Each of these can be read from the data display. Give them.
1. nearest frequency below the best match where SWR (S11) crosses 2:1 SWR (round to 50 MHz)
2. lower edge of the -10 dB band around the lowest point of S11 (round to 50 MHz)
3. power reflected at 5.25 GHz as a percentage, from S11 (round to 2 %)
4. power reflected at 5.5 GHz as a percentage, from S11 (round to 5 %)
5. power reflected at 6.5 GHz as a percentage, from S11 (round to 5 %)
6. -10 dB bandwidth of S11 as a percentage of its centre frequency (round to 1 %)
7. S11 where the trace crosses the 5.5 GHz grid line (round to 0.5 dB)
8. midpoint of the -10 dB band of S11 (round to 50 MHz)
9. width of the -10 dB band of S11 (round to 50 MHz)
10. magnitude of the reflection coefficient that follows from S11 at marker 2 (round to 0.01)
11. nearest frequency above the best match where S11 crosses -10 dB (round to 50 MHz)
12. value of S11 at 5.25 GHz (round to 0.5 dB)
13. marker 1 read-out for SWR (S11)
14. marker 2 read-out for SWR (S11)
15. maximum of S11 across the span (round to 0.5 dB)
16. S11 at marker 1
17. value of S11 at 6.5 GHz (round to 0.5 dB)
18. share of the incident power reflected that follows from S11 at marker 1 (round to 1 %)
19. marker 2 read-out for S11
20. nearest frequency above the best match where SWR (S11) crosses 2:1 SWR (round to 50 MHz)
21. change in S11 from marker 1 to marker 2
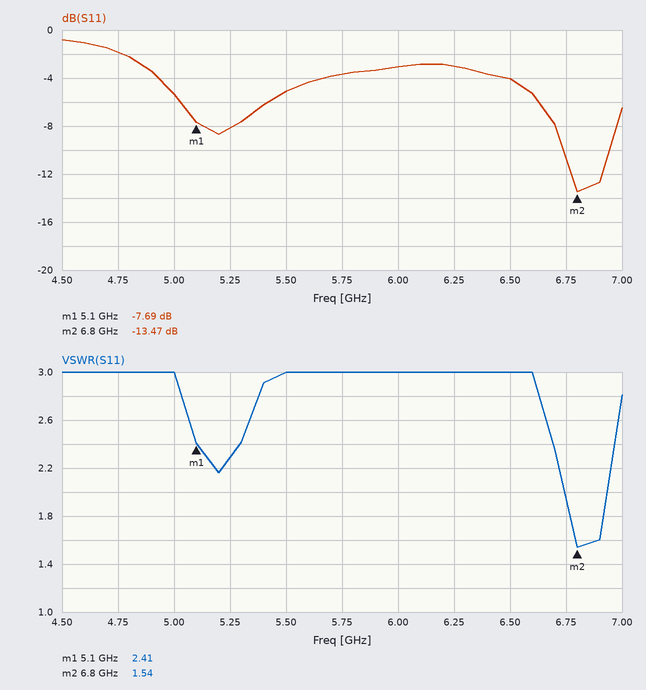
6.75 GHz
6.75 GHz
16 %
30 %
40 %
3 %
-5.0 dB
6.85 GHz
200 MHz
0.21
6.95 GHz
-8.0 dB
2.41
1.54
-1.0 dB
-7.69 dB
-4.0 dB
17 %
-13.47 dB
6.95 GHz
-5.78 dB
